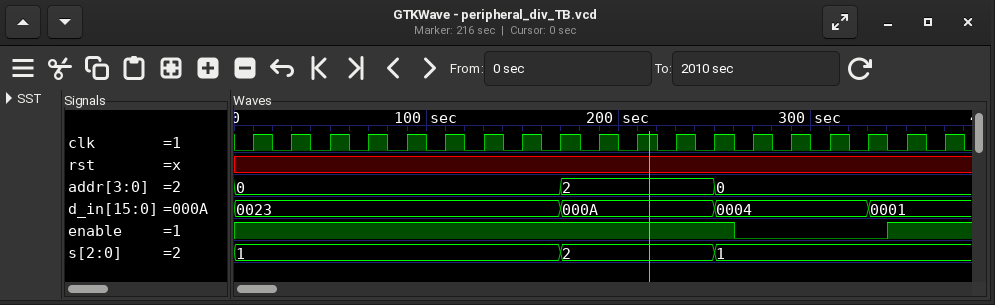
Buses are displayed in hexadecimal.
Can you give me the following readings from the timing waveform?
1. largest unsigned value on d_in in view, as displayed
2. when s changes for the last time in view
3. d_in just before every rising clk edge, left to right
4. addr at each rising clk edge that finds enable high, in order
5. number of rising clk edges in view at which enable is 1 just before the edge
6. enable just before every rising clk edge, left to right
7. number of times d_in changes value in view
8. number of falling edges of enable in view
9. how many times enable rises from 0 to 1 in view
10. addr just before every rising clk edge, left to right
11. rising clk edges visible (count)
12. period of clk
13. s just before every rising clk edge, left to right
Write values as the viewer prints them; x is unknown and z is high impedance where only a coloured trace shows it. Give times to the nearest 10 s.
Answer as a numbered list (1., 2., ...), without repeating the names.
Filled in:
1. 0023
2. 250 s
3. 0023, 0023, 0023, 0023, 0023, 0023, 0023, 0023, 0023, 000A, 000A, 000A, 000A, 0004, 0004, 0004, 0004, 0001, 0001
4. 0, 0, 0, 0, 0, 0, 0, 0, 0, 2, 2, 2, 2, 0, 0
5. 15
6. 1 1 1 1 1 1 1 1 1 1 1 1 1 0 0 0 0 1 1
7. 3
8. 1
9. 1
10. 0, 0, 0, 0, 0, 0, 0, 0, 0, 2, 2, 2, 2, 0, 0, 0, 0, 0, 0
11. 19
12. 20 s
13. 1, 1, 1, 1, 1, 1, 1, 1, 1, 2, 2, 2, 2, 1, 1, 1, 1, 1, 1
